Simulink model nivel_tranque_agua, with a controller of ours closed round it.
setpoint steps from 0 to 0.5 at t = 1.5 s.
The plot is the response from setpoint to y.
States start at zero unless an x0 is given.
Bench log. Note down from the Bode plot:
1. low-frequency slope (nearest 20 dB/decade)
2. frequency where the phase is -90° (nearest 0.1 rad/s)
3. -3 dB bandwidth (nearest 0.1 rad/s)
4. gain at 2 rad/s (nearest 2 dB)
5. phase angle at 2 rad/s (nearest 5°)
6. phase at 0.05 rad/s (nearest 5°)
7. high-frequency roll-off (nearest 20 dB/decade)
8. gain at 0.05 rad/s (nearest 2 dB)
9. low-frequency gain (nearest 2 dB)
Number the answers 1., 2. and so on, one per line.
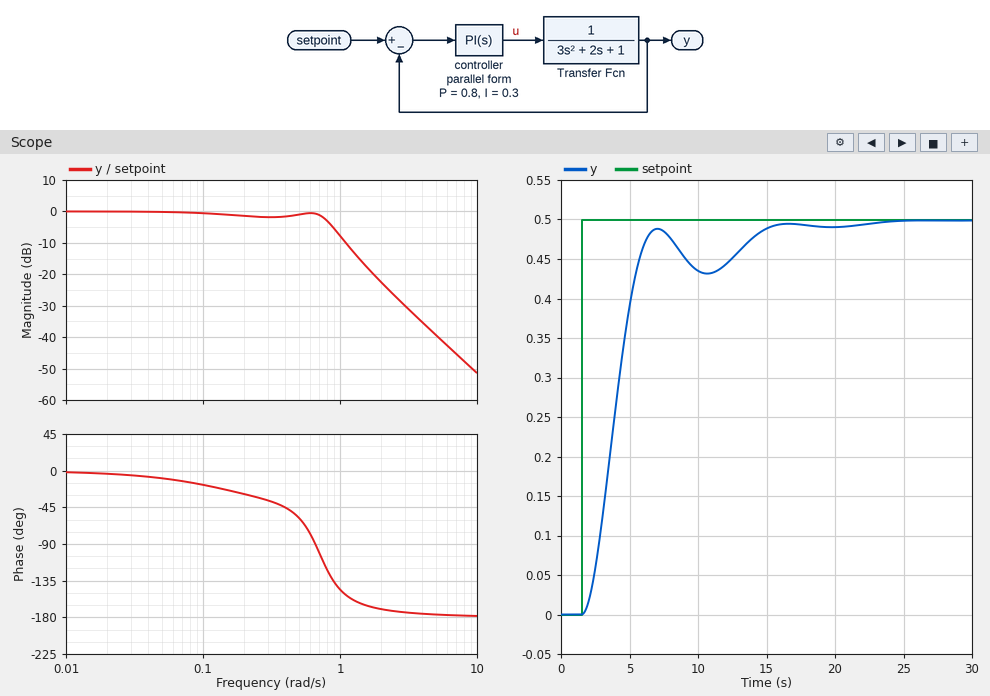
1. 0 dB/decade
2. 0.7 rad/s
3. 0.8 rad/s
4. -22 dB
5. -170°
6. -10°
7. -40 dB/decade
8. 0 dB
9. 0 dB
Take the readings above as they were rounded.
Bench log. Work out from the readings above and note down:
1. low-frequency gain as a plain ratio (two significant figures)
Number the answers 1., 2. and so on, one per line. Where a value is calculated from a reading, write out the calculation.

1. 10^(0 / 20) = 1.0
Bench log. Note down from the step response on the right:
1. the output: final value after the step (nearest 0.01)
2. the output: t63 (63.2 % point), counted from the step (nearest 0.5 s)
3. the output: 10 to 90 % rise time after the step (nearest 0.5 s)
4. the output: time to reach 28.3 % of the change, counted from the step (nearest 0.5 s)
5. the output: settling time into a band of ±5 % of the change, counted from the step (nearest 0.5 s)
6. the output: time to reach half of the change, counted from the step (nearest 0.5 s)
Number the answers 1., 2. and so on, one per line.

1. 0.50
2. 3.0 s
3. 3.5 s
4. 1.5 s
5. 12.5 s
6. 2.5 s
